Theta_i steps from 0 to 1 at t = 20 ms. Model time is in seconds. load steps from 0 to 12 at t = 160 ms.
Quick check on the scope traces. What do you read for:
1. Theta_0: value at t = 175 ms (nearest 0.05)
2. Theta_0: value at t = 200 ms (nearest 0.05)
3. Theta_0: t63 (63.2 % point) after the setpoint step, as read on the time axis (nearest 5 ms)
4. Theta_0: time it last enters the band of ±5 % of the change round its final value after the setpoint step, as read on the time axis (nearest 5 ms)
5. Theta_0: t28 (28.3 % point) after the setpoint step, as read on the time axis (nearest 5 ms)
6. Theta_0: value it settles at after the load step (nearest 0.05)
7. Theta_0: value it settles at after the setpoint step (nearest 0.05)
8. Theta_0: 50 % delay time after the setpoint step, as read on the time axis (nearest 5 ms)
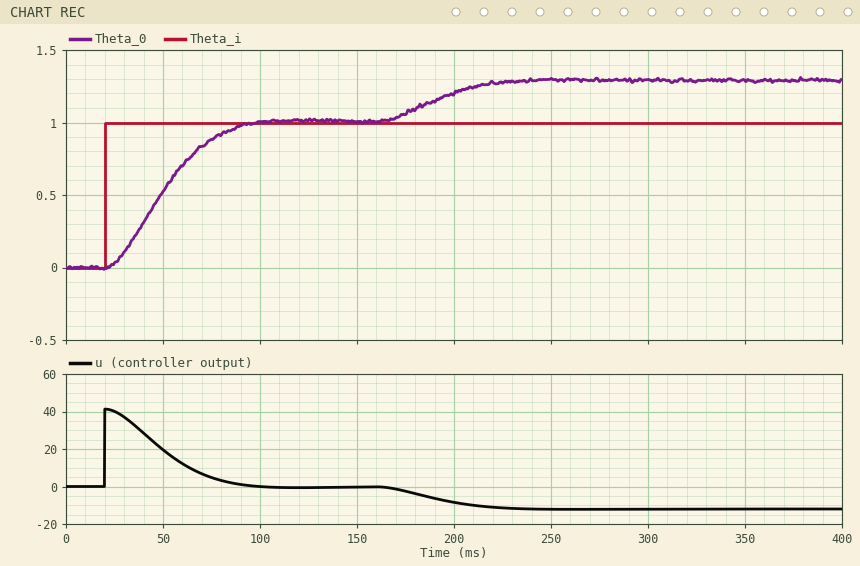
1.05
1.20
55 ms
85 ms
40 ms
1.30
1.00
50 ms
